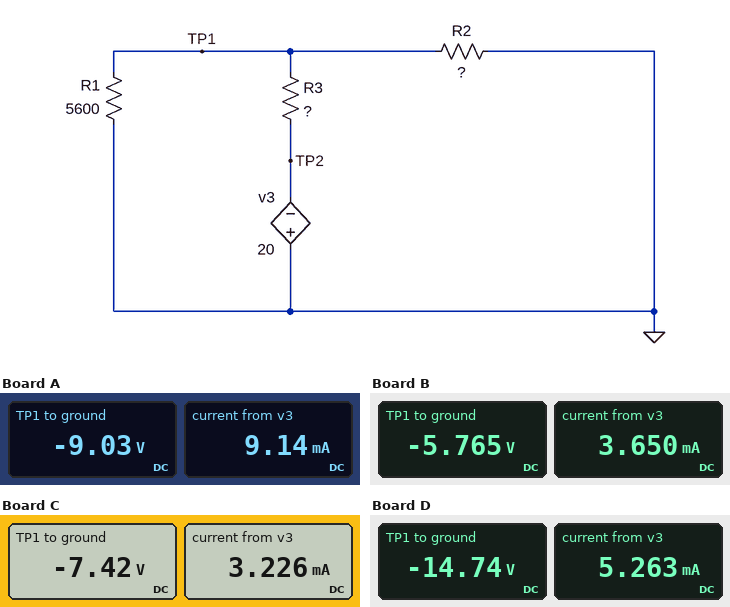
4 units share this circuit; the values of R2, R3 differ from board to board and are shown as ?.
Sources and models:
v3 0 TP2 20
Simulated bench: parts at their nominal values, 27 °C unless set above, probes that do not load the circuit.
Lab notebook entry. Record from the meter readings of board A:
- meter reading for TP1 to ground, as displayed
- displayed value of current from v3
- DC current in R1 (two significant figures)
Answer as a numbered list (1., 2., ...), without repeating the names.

1. -9.03 V
2. 9.14 mA
3. 1.6 mA
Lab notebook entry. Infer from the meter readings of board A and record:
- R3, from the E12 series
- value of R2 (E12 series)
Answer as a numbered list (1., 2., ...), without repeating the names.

1. 1.2 kΩ
2. 1.2 kΩ
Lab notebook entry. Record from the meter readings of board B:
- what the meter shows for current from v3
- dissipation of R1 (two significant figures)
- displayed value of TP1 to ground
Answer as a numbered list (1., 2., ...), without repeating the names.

1. 3.650 mA
2. 5.9 mW
3. -5.765 V
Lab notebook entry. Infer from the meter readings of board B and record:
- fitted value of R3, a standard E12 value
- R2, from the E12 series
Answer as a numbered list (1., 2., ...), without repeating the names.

1. 3.9 kΩ
2. 2.2 kΩ
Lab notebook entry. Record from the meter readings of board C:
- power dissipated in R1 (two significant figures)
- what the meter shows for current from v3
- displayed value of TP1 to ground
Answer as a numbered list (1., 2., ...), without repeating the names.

1. 9.8 mW
2. 3.226 mA
3. -7.42 V
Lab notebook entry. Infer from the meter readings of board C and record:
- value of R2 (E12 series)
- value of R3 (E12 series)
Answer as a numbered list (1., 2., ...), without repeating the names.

1. 3.9 kΩ
2. 3.9 kΩ
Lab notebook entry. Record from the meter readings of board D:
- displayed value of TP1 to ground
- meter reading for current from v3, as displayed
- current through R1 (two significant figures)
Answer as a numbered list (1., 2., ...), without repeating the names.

1. -14.74 V
2. 5.263 mA
3. 2.6 mA
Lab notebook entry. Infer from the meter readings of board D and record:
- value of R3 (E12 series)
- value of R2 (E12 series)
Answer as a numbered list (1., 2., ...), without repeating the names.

1. 1 kΩ
2. 5.6 kΩ
